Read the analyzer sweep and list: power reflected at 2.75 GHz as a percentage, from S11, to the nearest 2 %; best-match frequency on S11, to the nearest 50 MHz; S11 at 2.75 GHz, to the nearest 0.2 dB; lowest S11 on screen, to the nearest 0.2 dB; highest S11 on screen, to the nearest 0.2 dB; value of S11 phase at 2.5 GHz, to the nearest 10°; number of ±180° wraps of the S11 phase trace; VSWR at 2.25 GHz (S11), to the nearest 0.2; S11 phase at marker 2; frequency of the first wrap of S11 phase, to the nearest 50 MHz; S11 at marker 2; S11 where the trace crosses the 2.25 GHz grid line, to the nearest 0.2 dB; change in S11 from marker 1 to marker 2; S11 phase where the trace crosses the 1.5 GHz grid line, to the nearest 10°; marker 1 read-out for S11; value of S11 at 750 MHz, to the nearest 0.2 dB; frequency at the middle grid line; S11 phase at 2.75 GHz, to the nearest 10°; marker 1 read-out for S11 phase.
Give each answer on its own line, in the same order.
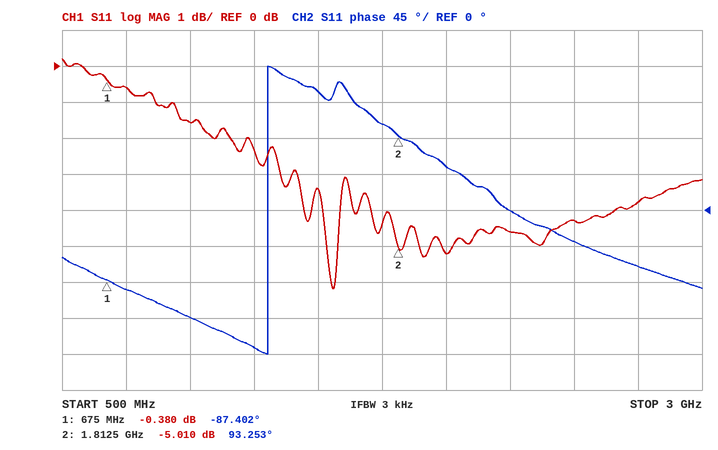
42 %
1.55 GHz
-3.8 dB
-6.2 dB
0.2 dB
-40°
1
3.8
93.253°
1.30 GHz
-5.010 dB
-4.6 dB
-4.630 dB
150°
-0.380 dB
-0.6 dB
1.75 GHz
-70°
-87.402°
